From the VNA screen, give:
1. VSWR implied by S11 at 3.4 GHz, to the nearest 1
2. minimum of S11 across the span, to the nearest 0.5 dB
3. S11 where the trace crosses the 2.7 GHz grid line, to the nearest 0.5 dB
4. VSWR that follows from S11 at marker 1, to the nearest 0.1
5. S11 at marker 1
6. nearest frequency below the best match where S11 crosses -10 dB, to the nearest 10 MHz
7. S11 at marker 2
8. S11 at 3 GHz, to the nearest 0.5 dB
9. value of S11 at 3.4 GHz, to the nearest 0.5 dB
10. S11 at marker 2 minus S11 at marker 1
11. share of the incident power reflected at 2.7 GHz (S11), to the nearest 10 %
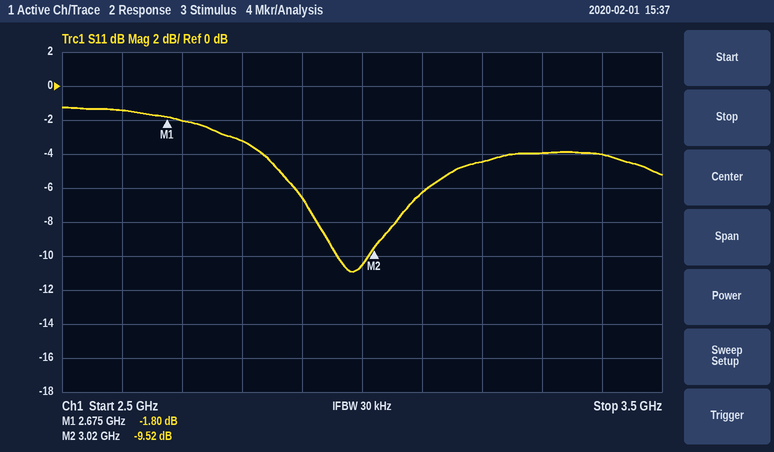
4
-11.0 dB
-2.0 dB
9.7
-1.80 dB
2.96 GHz
-9.52 dB
-10.5 dB
-4.0 dB
-7.72 dB
60 %
